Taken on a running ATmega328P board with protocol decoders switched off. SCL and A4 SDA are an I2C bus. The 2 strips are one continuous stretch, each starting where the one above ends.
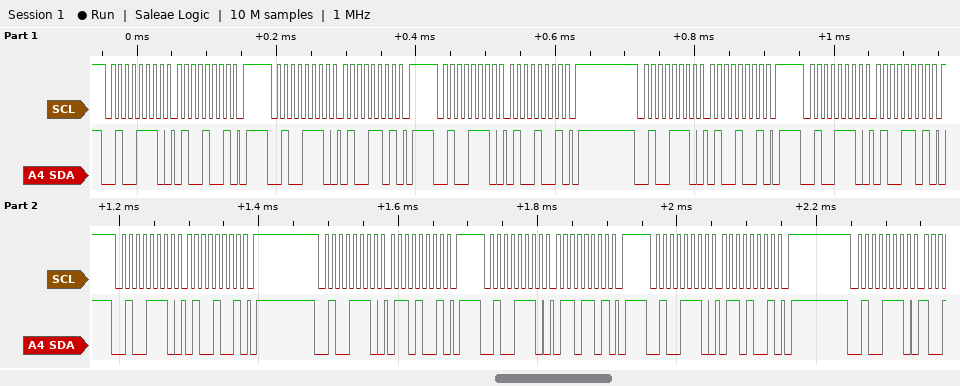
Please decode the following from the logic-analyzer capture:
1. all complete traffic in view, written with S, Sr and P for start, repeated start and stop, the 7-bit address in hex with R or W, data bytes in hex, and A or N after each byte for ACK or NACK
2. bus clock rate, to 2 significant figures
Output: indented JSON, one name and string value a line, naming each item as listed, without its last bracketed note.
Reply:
{
  "all complete traffic in view, written with S, Sr and P for start, repeated start and stop, the 7-bit address in hex with R or W, data bytes in hex, and A or N after each byte for ACK or NACK": "S 27W A 49 A P S 27W A 4D A P S 27W A 49 A P S 27W A 49 A P S 27W A 4D A P S 27W A 49 A P S 27W A 69 A P S 27W A 6D A P S 27W A 69 A P S 27W A",
  "bus clock rate, to 2 significant figures": "100 kHz"
}
